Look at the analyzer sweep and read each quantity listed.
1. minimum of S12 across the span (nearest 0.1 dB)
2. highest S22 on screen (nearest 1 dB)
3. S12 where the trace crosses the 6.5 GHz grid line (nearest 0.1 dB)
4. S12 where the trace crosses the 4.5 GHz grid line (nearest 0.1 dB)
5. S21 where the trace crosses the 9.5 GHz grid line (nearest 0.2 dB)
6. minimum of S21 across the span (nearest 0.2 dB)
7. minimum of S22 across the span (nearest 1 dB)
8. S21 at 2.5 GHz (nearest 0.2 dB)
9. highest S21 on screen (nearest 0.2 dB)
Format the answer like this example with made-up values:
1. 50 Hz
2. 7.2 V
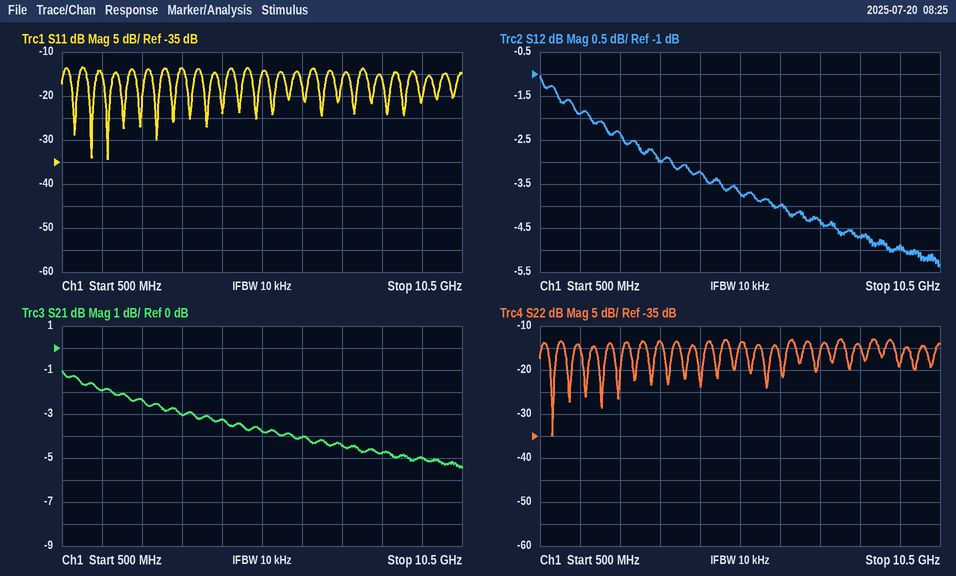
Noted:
1. -5.4 dB
2. -13 dB
3. -4.0 dB
4. -3.2 dB
5. -5.0 dB
6. -5.4 dB
7. -35 dB
8. -2.4 dB
9. -1.0 dB
